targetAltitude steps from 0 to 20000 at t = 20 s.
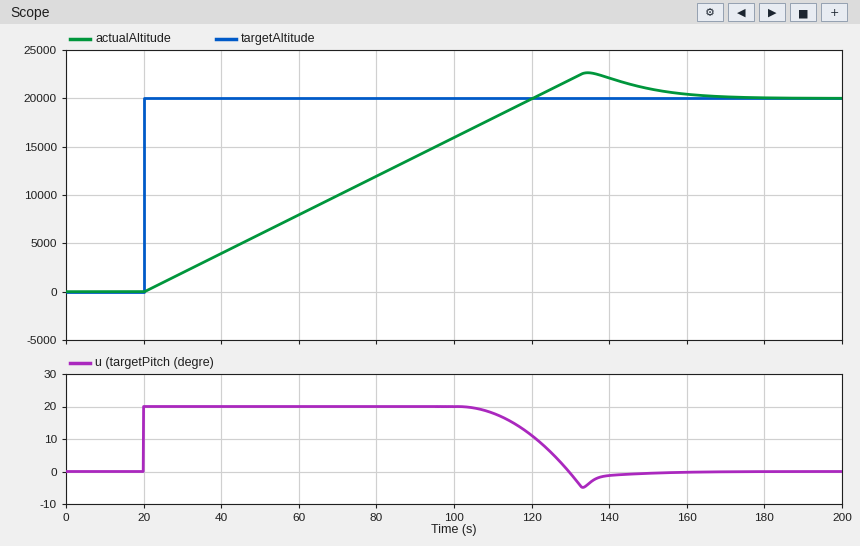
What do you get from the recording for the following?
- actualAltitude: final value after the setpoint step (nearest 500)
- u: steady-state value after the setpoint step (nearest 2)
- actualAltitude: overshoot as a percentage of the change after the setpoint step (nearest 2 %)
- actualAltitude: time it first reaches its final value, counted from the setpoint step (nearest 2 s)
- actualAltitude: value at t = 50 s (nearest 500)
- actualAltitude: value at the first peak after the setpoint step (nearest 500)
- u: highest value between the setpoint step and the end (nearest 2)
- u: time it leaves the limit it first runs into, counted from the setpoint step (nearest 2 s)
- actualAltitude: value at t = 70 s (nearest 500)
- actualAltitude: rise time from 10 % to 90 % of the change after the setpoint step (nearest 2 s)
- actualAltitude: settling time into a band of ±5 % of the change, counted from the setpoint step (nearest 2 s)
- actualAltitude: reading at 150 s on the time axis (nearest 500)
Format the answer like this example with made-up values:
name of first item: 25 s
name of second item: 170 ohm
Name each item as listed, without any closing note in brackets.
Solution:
actualAltitude: final value after the setpoint step: 20000
u: steady-state value after the setpoint step: 0
actualAltitude: overshoot as a percentage of the change after the setpoint step: 14 %
actualAltitude: time it first reaches its final value, counted from the setpoint step: 100 s
actualAltitude: value at t = 50 s: 6000
actualAltitude: value at the first peak after the setpoint step: 22500
u: highest value between the setpoint step and the end: 20
u: time it leaves the limit it first runs into, counted from the setpoint step: 84 s
actualAltitude: value at t = 70 s: 10000
actualAltitude: rise time from 10 % to 90 % of the change after the setpoint step: 80 s
actualAltitude: settling time into a band of ±5 % of the change, counted from the setpoint step: 130 s
actualAltitude: reading at 150 s on the time axis: 21000
